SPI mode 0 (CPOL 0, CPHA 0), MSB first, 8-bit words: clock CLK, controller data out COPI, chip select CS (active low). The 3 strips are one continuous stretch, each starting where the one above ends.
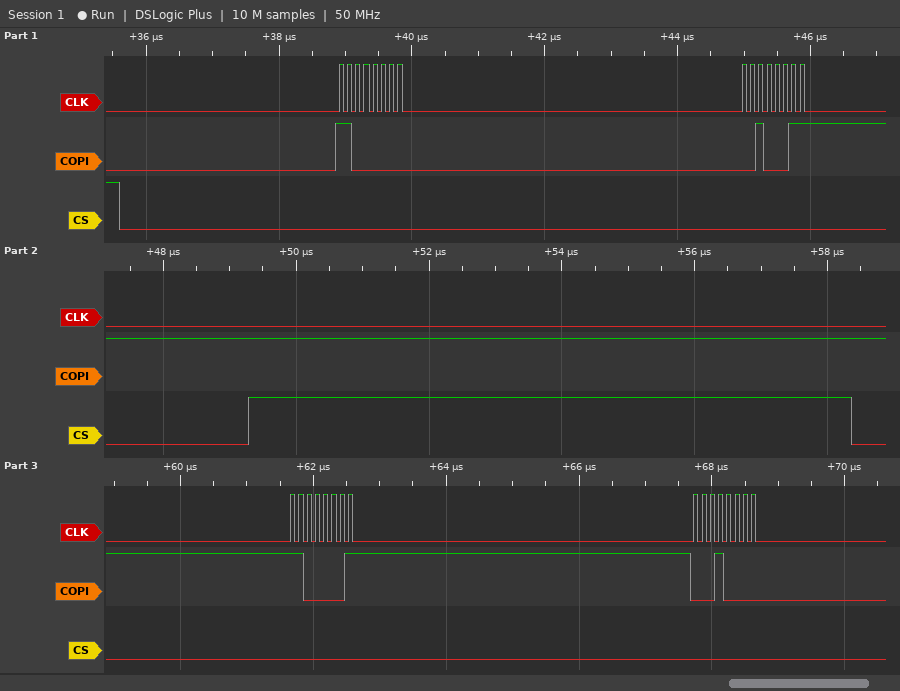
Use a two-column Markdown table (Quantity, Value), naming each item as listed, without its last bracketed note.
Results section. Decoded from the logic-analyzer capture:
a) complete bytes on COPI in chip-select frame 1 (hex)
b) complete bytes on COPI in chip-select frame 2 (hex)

| Quantity | Value |
|---|---|
| complete bytes on COPI in chip-select frame 1 | 0xC0 0x23 |
| complete bytes on COPI in chip-select frame 2 | 0xC1 0x10 |
